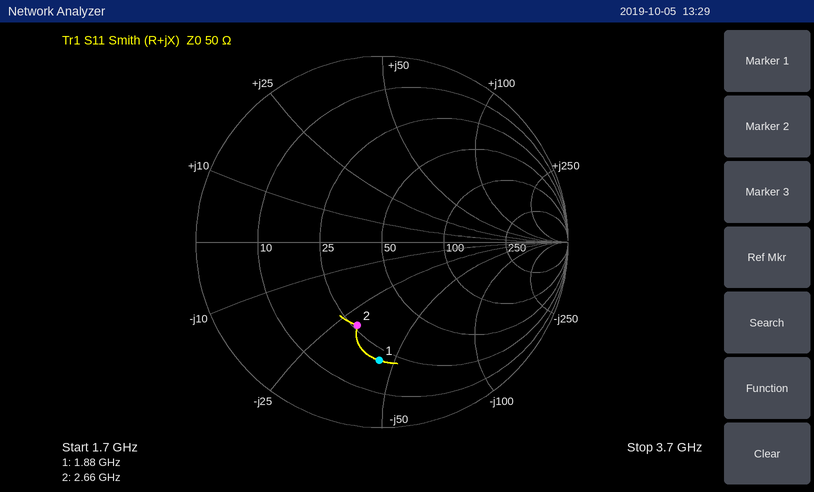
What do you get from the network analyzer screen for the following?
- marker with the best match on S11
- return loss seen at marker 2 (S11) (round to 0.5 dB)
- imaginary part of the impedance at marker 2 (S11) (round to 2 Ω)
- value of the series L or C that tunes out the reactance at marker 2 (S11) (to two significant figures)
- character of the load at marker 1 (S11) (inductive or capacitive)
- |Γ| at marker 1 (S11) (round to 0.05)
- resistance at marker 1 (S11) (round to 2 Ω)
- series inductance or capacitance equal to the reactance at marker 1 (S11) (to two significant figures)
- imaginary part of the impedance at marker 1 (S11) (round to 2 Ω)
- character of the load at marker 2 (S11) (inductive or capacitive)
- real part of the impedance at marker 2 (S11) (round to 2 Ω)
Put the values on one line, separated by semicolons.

marker 2; 6.5 dB; -30 Ω; 1.8 nH; capacitive; 0.65; 20 Ω; 1.9 pF; -44 Ω; capacitive; 26 Ω
